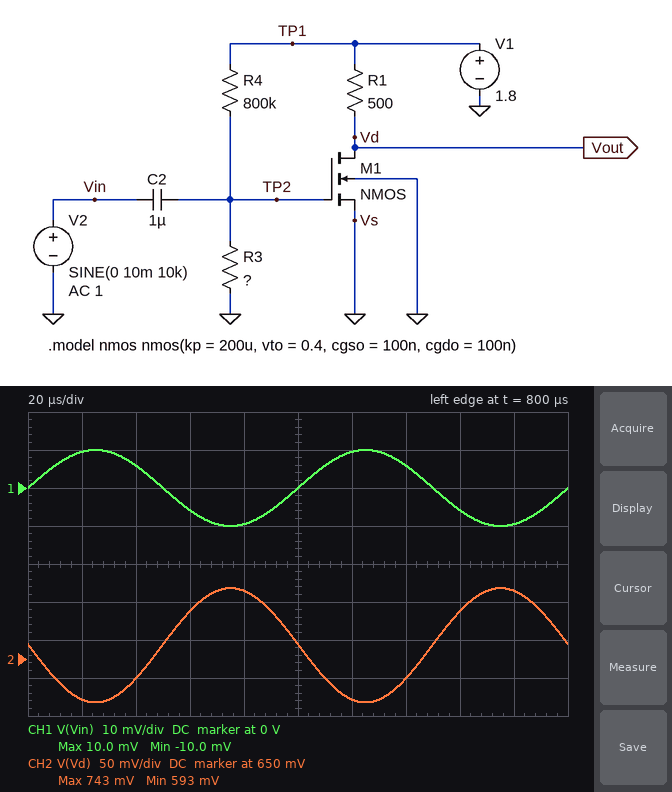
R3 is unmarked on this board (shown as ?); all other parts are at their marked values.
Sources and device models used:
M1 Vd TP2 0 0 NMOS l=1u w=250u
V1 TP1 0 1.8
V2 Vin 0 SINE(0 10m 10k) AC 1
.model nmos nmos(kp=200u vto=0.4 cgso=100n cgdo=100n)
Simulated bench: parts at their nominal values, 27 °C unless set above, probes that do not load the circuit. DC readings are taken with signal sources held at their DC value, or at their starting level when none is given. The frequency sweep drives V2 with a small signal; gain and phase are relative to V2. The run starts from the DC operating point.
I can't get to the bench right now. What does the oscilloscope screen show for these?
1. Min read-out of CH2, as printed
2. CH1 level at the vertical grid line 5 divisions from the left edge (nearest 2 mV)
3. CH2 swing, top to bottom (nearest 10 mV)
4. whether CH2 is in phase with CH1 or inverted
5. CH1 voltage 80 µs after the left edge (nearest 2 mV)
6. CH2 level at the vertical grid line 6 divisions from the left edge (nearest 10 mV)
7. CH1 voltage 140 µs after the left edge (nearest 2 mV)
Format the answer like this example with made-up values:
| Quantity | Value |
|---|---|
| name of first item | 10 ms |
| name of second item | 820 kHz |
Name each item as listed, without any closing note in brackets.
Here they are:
| Quantity | Value |
|---|---|
| Min read-out of CH2, as printed | 593 mV |
| CH1 level at the vertical grid line 5 divisions from the left edge | 0 V |
| CH2 swing, top to bottom | 150 mV |
| whether CH2 is in phase with CH1 or inverted | inverted |
| CH1 voltage 80 µs after the left edge | -10 mV |
| CH2 level at the vertical grid line 6 divisions from the left edge | 600 mV |
| CH1 voltage 140 µs after the left edge | 6 mV |
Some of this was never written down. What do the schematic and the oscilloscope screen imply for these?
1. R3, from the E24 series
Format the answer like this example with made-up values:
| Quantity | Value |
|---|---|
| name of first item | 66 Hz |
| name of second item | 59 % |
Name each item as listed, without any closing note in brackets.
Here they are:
| Quantity | Value |
|---|---|
| R3, from the E24 series | 510 kΩ |
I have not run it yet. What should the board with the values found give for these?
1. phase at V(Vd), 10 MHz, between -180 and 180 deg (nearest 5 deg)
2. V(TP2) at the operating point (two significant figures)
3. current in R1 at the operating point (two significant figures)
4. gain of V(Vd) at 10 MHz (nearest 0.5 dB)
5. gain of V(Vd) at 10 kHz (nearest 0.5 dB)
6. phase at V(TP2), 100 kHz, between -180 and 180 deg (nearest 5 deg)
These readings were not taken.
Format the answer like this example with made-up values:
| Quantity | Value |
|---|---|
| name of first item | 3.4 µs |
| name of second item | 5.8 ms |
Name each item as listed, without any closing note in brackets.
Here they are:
| Quantity | Value |
|---|---|
| phase at V(Vd), 10 MHz, between -180 and 180 deg | 135 deg |
| V(TP2) at the operating point | 700 mV |
| current in R1 at the operating point | 2.3 mA |
| gain of V(Vd) at 10 MHz | 15.5 dB |
| gain of V(Vd) at 10 kHz | 17.5 dB |
| phase at V(TP2), 100 kHz, between -180 and 180 deg | 0 deg |
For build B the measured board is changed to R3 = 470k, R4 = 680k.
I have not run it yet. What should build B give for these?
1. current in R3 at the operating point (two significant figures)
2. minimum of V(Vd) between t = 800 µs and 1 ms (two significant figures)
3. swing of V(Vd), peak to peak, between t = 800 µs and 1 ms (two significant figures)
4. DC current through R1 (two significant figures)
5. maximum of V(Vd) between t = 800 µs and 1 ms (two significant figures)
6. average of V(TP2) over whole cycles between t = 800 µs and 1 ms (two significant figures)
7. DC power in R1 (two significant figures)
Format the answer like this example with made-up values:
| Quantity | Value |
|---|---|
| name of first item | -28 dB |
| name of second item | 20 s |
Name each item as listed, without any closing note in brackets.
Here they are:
| Quantity | Value |
|---|---|
| current in R3 at the operating point | 1.6 µA |
| minimum of V(Vd) between t = 800 µs and 1 ms | 320 mV |
| swing of V(Vd), peak to peak, between t = 800 µs and 1 ms | 160 mV |
| DC current through R1 | 2.8 mA |
| maximum of V(Vd) between t = 800 µs and 1 ms | 470 mV |
| average of V(TP2) over whole cycles between t = 800 µs and 1 ms | 740 mV |
| DC power in R1 | 4.0 mW |
